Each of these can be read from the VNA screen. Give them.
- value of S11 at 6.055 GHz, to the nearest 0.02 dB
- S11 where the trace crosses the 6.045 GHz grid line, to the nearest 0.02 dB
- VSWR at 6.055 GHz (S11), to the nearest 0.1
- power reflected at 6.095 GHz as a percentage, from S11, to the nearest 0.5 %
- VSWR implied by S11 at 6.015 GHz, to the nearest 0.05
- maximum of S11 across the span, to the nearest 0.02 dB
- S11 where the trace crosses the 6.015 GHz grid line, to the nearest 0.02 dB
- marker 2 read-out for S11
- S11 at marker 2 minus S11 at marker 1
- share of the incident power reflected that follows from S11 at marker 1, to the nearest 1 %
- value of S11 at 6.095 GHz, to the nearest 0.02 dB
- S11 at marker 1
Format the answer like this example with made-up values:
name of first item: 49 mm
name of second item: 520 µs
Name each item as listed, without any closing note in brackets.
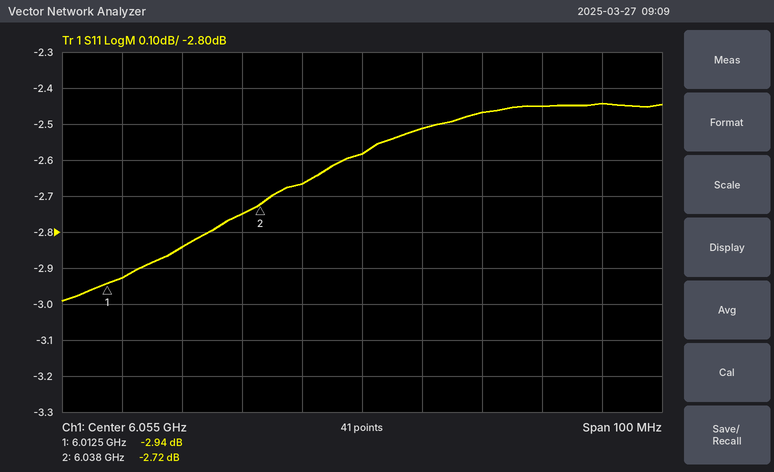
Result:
value of S11 at 6.055 GHz, to the nearest 0.02 dB: -2.58 dB
S11 where the trace crosses the 6.045 GHz grid line, to the nearest 0.02 dB: -2.66 dB
VSWR at 6.055 GHz (S11), to the nearest 0.1: 6.8
power reflected at 6.095 GHz as a percentage, from S11, to the nearest 0.5 %: 57.0 %
VSWR implied by S11 at 6.015 GHz, to the nearest 0.05: 6.00
maximum of S11 across the span, to the nearest 0.02 dB: -2.44 dB
S11 where the trace crosses the 6.015 GHz grid line, to the nearest 0.02 dB: -2.92 dB
marker 2 read-out for S11: -2.72 dB
S11 at marker 2 minus S11 at marker 1: 0.22 dB
share of the incident power reflected that follows from S11 at marker 1, to the nearest 1 %: 51 %
value of S11 at 6.095 GHz, to the nearest 0.02 dB: -2.44 dB
S11 at marker 1: -2.94 dB
